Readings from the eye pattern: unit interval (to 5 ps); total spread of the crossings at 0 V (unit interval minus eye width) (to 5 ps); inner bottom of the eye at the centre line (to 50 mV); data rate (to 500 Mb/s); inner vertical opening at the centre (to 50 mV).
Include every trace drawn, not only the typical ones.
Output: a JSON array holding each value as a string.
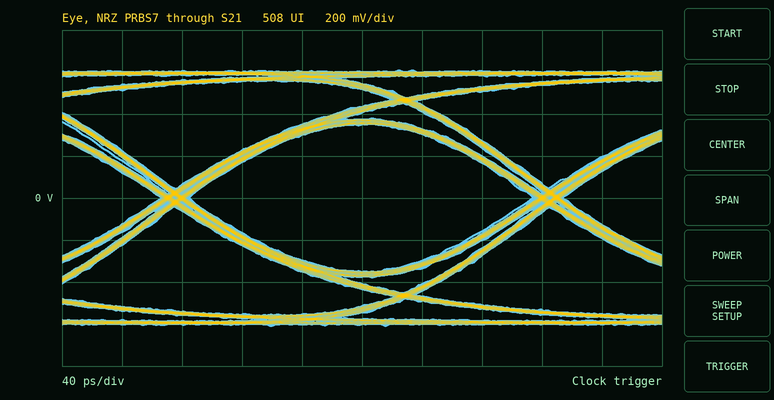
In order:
["250 ps", "20 ps", "-350 mV", "4.0 Gb/s", "700 mV"]
